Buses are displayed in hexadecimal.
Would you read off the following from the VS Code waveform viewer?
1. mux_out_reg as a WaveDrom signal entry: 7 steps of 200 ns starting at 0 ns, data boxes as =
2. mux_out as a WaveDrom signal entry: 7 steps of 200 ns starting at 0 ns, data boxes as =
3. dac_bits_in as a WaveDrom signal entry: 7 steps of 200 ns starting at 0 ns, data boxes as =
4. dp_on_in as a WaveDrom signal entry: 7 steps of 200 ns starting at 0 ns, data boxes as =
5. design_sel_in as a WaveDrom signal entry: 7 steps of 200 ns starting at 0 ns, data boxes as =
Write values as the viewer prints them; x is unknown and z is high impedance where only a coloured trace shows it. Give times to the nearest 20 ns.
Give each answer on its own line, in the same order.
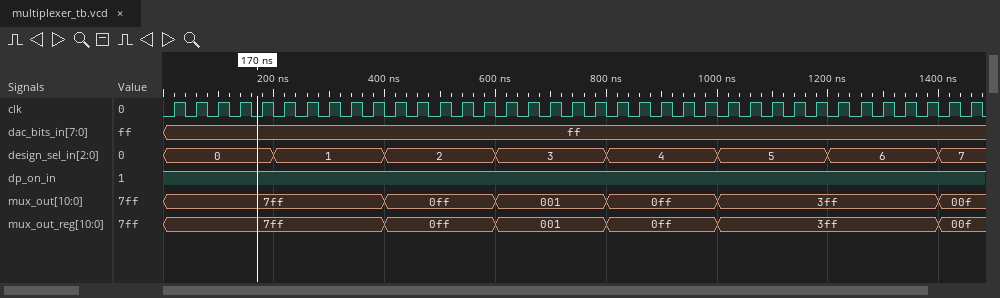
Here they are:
{name: 'mux_out_reg', wave: '=.====.', data: '7ff 0ff 001 0ff 3ff'}
{name: 'mux_out', wave: '=.====.', data: '7ff 0ff 001 0ff 3ff'}
{name: 'dac_bits_in', wave: '=......', data: 'ff'}
{name: 'dp_on_in', wave: '1......'}
{name: 'design_sel_in', wave: '=======', data: '0 1 2 3 4 5 6'}
